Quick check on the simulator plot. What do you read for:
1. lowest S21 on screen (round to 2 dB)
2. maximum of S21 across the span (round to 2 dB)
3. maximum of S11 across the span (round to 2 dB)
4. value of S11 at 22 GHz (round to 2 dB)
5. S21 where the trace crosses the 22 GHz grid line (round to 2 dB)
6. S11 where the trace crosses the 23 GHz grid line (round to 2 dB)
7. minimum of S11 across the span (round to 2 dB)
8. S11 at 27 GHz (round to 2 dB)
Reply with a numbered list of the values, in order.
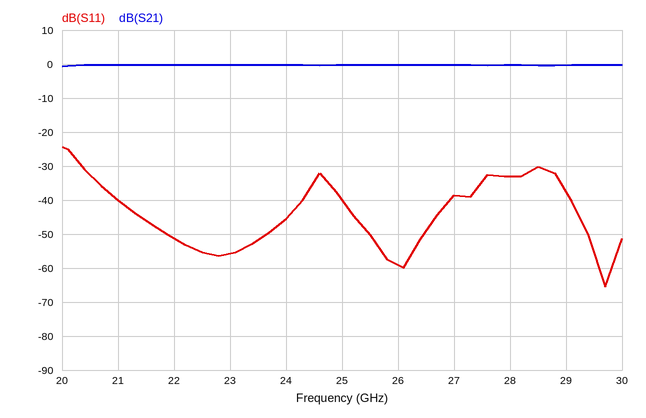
1. 0 dB
2. 0 dB
3. -24 dB
4. -52 dB
5. 0 dB
6. -56 dB
7. -66 dB
8. -38 dB
